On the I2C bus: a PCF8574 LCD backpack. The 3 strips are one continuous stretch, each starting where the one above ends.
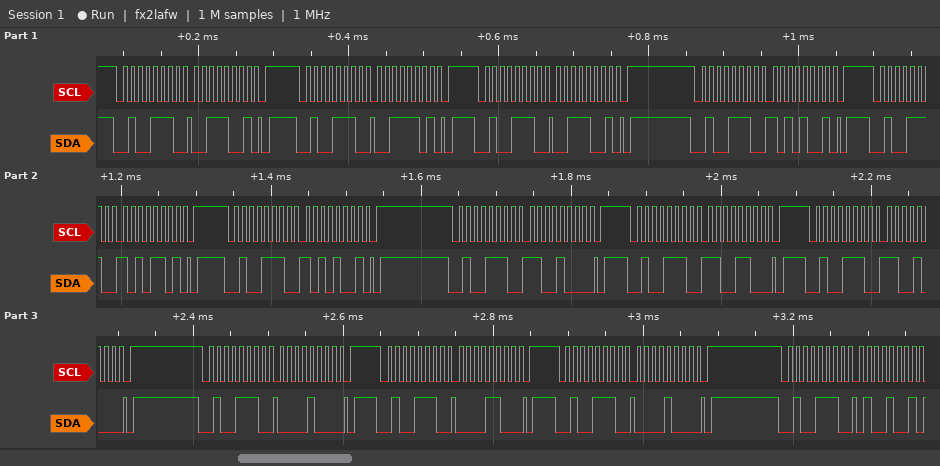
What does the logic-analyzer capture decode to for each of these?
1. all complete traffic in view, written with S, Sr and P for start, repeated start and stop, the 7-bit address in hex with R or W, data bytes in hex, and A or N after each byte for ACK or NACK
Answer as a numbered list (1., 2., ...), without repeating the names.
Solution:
1. S 27W A 39 A P S 27W A 3D A P S 27W A 39 A P S 27W A A9 A P S 27W A AD A P S 27W A A9 A P S 27W A C8 A P S 27W A CC A P S 27W A C8 A P S 27W A 08 A P S 27W A 0C A P S 27W A 08 A P S 27W A 49 A
